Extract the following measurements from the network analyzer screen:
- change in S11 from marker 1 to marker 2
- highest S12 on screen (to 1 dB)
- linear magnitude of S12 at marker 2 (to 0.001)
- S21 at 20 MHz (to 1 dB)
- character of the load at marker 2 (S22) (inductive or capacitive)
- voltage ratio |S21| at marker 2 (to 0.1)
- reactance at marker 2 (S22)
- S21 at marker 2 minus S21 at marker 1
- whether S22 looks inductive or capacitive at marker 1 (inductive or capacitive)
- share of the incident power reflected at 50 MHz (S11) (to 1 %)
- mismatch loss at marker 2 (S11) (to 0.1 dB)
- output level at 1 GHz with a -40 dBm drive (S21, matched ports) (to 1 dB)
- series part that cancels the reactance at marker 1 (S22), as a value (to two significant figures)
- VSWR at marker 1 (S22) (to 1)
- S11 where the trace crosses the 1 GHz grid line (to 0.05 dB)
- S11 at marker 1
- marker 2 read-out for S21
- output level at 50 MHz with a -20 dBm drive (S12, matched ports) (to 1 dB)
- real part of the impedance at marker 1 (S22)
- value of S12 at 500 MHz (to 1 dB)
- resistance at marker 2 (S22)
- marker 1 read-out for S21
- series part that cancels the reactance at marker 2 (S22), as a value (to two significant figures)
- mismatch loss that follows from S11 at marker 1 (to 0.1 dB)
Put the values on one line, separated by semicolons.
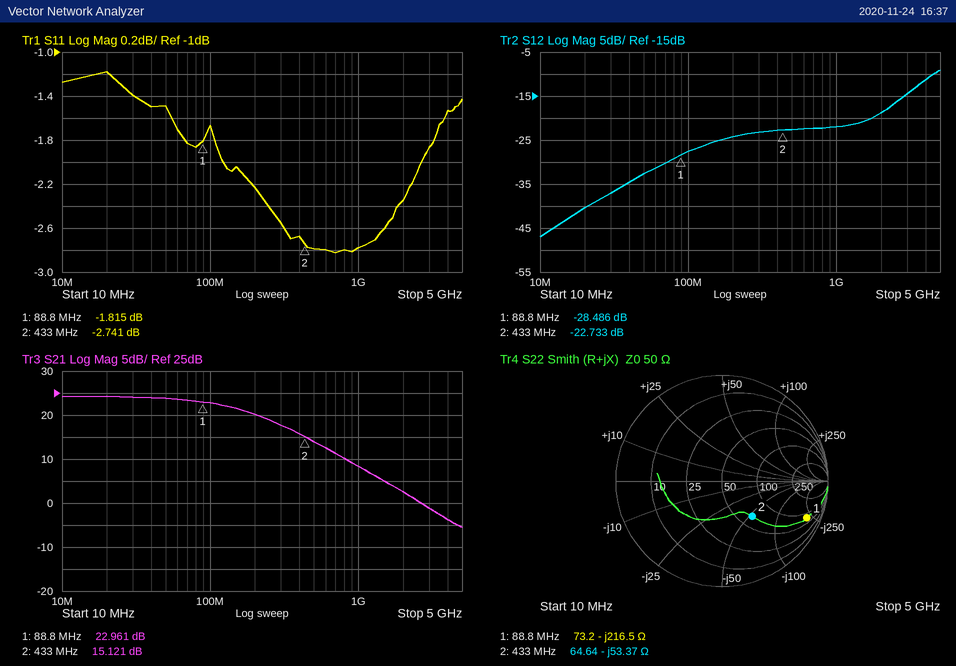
-0.926 dB; -9 dB; 0.073; 24 dB; capacitive; 5.7; -53.37 Ω; -7.840 dB; capacitive; 71 %; 3.3 dB; -32 dBm; 390 nH; 15; -2.80 dB; -1.815 dB; 15.121 dB; -53 dBm; 73.2 Ω; -23 dB; 64.64 Ω; 22.961 dB; 20 nH; 4.7 dB
